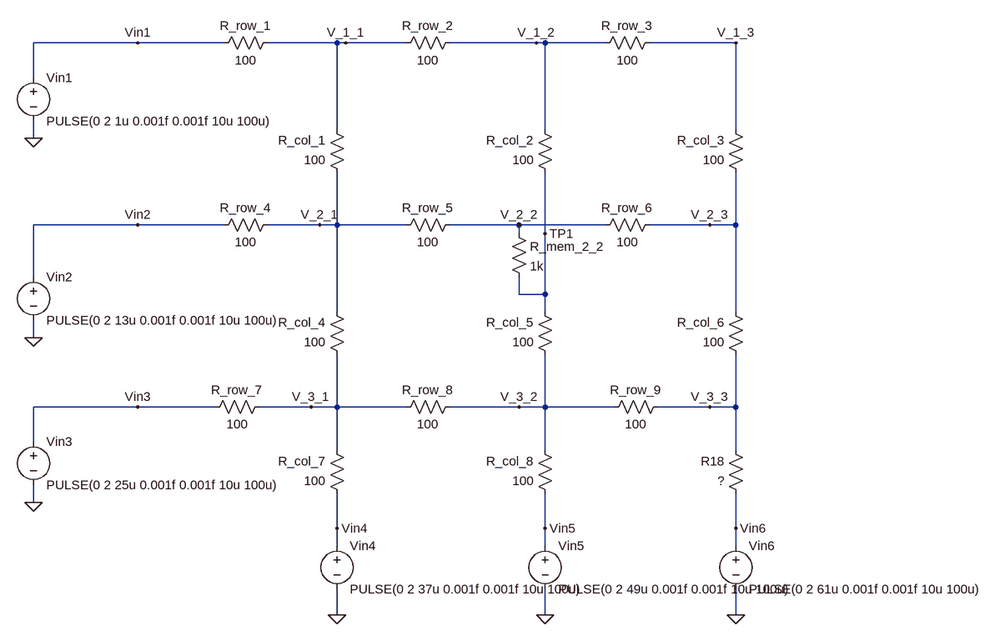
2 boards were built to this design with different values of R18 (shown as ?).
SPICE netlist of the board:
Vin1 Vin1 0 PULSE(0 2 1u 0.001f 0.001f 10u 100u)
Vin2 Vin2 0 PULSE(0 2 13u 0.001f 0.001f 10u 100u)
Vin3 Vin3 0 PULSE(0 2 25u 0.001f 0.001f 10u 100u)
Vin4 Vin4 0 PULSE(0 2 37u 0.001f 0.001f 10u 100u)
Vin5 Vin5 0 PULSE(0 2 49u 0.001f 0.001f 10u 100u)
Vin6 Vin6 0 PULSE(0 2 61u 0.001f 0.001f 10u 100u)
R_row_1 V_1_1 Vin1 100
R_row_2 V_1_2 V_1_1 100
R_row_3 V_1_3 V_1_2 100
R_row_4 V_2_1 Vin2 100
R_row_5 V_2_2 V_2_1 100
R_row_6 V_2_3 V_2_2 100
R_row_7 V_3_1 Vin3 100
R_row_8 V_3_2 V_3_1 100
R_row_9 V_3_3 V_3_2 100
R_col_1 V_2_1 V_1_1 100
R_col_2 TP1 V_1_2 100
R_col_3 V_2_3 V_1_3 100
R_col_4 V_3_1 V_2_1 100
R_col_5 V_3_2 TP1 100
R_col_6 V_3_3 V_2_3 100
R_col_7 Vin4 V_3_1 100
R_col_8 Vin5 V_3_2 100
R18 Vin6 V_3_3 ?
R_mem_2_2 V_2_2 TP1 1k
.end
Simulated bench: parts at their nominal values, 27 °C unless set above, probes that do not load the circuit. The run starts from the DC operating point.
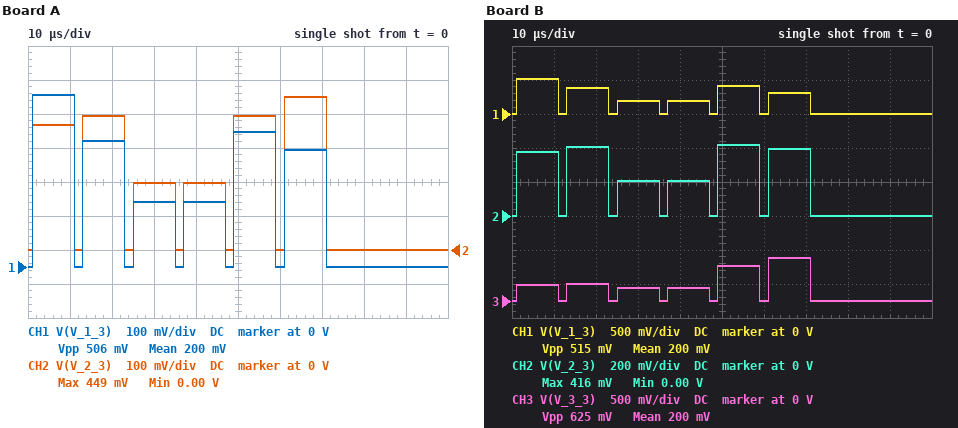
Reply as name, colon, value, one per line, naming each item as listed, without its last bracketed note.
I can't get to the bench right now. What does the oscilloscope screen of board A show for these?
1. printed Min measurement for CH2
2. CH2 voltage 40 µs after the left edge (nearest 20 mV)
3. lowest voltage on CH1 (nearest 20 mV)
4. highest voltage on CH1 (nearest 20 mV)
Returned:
printed Min measurement for CH2: 0.00 V
CH2 voltage 40 µs after the left edge: 200 mV
lowest voltage on CH1: 0 V
highest voltage on CH1: 500 mV
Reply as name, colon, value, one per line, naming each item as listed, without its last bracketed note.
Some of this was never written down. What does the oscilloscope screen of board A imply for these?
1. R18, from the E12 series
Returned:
R18, from the E12 series: 180 Ω
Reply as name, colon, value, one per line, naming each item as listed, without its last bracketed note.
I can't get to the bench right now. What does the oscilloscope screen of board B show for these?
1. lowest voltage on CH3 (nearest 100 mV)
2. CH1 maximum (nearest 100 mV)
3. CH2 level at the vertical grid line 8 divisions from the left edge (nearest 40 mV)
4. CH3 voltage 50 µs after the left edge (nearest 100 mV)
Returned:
lowest voltage on CH3: 0 V
CH1 maximum: 500 mV
CH2 level at the vertical grid line 8 divisions from the left edge: 0 V
CH3 voltage 50 µs after the left edge: 500 mV
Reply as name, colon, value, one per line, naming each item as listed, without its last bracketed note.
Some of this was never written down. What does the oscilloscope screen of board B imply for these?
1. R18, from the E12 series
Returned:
R18, from the E12 series: 220 Ω
